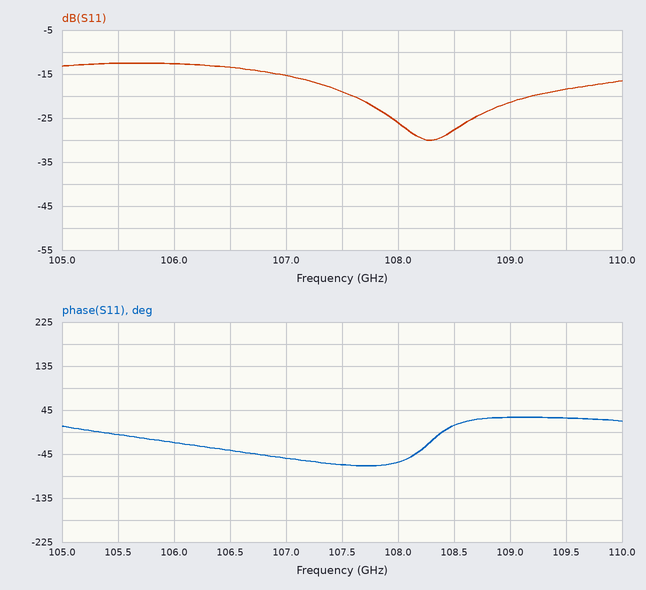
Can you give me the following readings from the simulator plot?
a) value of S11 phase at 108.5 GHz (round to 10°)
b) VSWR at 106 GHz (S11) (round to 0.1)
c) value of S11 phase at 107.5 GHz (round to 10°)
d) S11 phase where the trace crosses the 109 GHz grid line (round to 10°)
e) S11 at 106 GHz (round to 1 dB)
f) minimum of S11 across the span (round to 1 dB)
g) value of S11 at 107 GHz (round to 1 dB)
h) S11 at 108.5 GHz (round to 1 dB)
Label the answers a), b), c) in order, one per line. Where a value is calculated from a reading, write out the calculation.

a) 10°
b) |Γ| = 10^(-13/20) = 0.2239; VSWR = (1 + 0.2239)/(1 − 0.2239) ≈ 1.6
c) -70°
d) 30°
e) -13 dB
f) -30 dB
g) -15 dB
h) -28 dB
